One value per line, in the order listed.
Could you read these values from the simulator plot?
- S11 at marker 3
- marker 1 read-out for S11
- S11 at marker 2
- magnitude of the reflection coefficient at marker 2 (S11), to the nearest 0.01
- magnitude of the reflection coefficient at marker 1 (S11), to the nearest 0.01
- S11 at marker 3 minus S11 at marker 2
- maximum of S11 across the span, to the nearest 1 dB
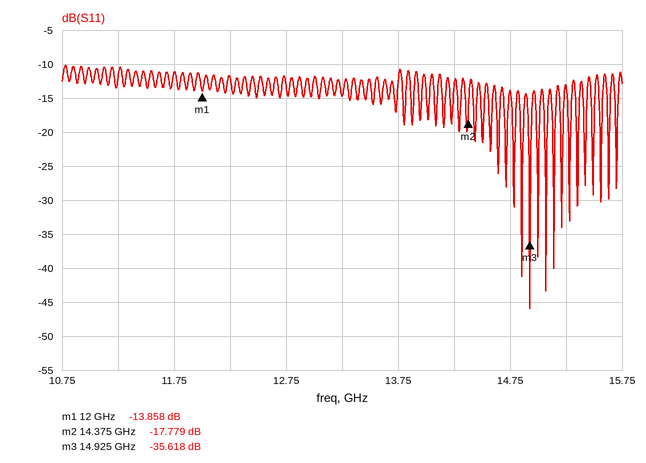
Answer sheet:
-35.618 dB
-13.858 dB
-17.779 dB
0.13
0.20
-17.839 dB
-10 dB
